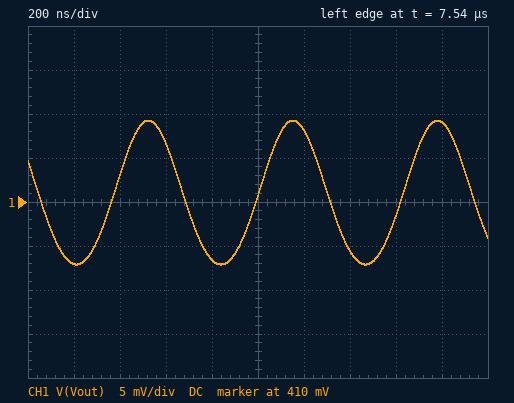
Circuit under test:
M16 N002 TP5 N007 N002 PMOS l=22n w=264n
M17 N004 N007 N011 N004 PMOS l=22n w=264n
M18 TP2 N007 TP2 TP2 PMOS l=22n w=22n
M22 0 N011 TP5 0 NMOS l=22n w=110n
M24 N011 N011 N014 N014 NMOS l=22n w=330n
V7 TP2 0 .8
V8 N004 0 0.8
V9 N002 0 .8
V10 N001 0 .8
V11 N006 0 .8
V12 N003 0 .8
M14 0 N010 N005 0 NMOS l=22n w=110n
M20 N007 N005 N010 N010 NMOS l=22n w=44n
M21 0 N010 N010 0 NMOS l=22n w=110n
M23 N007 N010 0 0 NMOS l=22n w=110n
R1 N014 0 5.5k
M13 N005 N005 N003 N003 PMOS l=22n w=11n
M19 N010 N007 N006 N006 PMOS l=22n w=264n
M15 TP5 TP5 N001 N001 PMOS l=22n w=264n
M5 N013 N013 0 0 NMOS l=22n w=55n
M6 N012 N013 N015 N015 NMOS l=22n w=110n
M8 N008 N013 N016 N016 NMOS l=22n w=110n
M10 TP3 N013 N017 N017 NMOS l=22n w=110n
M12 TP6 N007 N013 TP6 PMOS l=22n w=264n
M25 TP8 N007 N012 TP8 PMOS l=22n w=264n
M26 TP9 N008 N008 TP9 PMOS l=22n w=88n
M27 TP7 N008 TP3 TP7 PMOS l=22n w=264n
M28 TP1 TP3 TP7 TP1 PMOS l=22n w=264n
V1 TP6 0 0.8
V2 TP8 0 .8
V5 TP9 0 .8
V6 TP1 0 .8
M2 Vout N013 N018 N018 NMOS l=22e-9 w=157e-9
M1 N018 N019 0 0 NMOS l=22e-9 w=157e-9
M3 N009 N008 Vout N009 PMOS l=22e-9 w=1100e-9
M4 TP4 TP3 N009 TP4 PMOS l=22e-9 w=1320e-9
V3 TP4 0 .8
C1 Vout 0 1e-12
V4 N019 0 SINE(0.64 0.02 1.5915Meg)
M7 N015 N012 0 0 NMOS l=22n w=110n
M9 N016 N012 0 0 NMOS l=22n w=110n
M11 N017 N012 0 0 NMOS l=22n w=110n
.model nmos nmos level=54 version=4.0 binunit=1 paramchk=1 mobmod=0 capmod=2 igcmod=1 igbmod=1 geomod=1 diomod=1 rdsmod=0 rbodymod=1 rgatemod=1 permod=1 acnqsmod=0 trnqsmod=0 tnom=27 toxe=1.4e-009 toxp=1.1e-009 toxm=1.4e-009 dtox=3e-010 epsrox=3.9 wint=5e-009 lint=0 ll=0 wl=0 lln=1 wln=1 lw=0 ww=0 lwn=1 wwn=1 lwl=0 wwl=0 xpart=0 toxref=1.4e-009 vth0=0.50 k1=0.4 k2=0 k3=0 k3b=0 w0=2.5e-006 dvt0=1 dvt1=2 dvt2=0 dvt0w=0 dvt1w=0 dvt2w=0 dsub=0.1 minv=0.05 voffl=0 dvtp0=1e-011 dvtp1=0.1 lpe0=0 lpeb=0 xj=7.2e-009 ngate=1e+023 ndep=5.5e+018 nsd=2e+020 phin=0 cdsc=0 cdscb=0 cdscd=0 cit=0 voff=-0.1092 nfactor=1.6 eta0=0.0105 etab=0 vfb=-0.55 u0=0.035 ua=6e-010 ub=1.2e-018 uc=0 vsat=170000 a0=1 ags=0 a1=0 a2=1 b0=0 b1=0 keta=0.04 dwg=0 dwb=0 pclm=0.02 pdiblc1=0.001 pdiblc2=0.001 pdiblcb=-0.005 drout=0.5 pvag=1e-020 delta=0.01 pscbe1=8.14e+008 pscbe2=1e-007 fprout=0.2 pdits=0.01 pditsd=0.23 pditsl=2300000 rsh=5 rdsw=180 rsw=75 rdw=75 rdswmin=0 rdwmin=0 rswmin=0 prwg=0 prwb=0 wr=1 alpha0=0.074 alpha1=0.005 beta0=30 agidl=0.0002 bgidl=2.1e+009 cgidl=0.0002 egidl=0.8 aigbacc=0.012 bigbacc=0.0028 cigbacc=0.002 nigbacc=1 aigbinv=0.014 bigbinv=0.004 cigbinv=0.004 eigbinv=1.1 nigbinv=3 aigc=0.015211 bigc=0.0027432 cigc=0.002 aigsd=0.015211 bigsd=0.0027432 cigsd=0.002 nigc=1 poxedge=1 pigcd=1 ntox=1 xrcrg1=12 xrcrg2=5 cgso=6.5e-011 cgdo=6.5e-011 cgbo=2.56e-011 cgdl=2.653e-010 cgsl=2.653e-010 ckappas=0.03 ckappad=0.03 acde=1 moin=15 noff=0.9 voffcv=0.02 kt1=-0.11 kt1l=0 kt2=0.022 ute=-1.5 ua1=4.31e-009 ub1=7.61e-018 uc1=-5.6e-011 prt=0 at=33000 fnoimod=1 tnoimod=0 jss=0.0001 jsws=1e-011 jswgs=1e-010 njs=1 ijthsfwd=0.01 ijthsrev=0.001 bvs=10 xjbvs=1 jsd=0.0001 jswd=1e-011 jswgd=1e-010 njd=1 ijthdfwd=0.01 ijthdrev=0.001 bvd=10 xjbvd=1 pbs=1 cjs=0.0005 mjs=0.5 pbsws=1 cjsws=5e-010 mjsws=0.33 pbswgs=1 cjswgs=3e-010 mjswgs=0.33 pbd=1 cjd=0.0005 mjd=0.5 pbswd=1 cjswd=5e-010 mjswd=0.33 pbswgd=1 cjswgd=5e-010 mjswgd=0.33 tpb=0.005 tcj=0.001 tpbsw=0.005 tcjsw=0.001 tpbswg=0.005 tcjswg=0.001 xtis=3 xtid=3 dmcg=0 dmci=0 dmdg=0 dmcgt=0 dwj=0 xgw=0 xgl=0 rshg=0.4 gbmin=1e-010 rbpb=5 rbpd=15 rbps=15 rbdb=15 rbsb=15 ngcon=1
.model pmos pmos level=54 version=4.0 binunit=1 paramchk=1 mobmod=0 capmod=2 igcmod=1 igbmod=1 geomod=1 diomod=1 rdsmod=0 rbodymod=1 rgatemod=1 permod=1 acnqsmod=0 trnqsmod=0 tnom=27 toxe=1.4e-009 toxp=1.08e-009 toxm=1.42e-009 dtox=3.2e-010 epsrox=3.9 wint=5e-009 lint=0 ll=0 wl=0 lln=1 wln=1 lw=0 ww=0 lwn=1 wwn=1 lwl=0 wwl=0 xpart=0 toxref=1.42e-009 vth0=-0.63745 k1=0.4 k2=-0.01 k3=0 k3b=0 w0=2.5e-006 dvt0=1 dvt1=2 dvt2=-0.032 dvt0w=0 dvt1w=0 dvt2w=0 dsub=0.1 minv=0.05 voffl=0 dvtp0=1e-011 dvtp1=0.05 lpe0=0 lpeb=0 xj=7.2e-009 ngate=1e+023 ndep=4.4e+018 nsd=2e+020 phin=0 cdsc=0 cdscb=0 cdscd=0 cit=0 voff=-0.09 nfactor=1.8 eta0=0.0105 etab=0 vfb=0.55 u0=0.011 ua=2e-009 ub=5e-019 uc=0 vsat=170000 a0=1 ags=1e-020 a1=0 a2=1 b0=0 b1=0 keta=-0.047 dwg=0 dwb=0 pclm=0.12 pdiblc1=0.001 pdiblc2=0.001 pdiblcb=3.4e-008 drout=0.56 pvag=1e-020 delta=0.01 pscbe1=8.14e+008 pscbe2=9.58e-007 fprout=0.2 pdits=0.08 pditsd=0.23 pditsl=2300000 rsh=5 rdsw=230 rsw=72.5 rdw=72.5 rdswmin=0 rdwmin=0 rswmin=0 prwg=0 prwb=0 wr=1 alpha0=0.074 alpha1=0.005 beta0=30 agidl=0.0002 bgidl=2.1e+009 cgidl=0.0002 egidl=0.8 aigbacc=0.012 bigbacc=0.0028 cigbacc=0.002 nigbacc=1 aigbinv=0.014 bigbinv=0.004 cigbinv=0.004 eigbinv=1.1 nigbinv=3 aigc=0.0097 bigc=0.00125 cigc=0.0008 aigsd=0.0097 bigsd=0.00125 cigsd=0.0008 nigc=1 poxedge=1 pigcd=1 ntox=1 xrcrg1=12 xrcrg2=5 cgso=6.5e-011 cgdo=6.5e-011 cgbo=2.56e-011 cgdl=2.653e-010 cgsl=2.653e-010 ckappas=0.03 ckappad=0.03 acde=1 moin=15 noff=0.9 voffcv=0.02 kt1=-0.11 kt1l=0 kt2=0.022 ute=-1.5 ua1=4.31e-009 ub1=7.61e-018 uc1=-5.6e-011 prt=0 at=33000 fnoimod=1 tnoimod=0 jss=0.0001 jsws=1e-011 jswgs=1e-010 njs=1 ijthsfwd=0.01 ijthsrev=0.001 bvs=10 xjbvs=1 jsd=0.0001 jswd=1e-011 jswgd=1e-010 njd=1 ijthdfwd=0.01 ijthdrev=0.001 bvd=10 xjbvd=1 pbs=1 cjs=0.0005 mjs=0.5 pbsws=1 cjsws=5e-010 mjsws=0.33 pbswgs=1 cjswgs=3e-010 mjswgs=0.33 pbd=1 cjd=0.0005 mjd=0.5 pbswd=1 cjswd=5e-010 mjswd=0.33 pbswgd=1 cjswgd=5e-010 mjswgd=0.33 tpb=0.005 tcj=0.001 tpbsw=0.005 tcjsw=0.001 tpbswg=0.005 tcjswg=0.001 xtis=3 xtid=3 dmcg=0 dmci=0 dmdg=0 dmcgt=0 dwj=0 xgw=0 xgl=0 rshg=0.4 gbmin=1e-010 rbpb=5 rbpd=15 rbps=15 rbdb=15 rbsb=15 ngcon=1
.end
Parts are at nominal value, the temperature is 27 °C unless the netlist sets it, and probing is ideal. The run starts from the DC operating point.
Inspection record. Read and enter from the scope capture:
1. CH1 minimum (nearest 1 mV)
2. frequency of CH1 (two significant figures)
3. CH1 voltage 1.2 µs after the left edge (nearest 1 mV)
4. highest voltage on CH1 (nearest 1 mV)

403 mV
1.6 MHz
418 mV
419 mV
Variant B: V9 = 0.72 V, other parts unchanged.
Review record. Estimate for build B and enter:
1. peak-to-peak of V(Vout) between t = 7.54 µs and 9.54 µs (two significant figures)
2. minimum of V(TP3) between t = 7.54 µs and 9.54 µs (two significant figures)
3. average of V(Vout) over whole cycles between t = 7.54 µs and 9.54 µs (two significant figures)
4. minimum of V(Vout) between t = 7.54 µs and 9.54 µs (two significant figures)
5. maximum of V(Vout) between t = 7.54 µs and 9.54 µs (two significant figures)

51 mV
77 mV
480 mV
460 mV
510 mV
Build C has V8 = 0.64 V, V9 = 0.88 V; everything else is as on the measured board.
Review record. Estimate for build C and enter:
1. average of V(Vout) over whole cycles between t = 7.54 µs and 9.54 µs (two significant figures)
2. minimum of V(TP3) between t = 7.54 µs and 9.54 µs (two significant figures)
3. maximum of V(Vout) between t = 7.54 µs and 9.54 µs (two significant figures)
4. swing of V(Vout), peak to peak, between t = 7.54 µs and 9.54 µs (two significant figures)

470 mV
91 mV
490 mV
36 mV
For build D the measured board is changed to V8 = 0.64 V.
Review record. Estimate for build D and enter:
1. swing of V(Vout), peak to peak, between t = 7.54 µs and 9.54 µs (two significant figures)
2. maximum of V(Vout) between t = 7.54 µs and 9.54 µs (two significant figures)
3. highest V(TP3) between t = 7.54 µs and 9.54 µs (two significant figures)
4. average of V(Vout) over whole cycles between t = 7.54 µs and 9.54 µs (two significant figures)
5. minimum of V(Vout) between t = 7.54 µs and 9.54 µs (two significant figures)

53 mV
510 mV
76 mV
480 mV
460 mV
